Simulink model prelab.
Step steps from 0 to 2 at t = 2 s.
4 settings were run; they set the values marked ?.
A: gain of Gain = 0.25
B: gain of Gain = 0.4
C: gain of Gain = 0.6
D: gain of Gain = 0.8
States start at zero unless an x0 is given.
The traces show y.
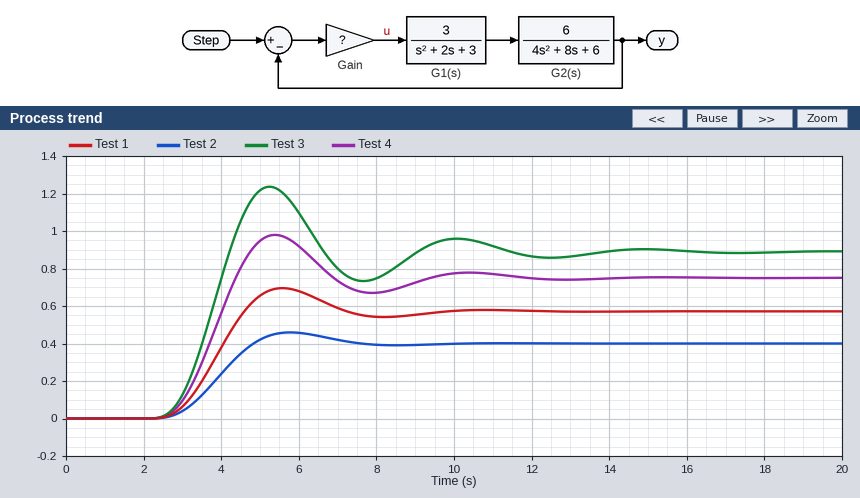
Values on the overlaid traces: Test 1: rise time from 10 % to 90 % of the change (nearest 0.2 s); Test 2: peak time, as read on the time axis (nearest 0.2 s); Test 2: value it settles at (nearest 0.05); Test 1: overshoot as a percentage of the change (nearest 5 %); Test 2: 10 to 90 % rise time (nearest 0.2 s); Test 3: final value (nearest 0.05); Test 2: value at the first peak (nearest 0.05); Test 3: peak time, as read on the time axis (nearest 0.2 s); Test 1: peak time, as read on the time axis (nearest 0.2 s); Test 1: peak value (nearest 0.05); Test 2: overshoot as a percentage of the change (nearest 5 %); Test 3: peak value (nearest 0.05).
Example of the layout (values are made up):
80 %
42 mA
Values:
1.4 s
5.8 s
0.40
20 %
1.6 s
0.90
0.45
5.2 s
5.6 s
0.70
15 %
1.25
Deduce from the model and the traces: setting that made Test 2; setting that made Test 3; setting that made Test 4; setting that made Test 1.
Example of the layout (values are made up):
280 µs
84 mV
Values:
A
D
C
B
